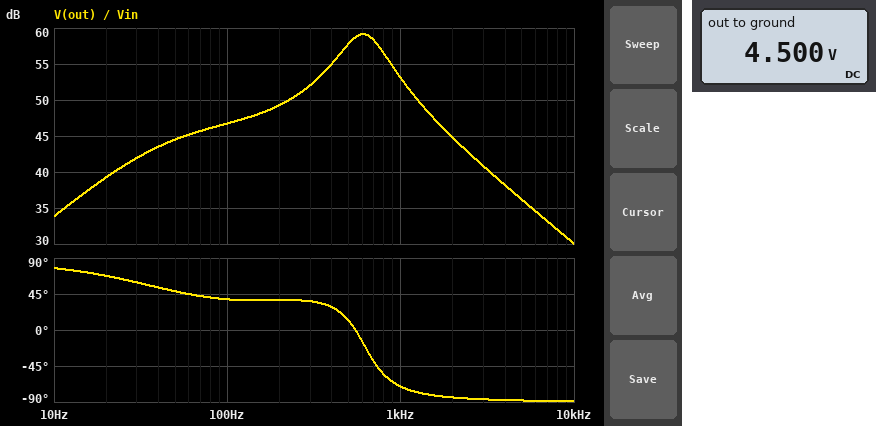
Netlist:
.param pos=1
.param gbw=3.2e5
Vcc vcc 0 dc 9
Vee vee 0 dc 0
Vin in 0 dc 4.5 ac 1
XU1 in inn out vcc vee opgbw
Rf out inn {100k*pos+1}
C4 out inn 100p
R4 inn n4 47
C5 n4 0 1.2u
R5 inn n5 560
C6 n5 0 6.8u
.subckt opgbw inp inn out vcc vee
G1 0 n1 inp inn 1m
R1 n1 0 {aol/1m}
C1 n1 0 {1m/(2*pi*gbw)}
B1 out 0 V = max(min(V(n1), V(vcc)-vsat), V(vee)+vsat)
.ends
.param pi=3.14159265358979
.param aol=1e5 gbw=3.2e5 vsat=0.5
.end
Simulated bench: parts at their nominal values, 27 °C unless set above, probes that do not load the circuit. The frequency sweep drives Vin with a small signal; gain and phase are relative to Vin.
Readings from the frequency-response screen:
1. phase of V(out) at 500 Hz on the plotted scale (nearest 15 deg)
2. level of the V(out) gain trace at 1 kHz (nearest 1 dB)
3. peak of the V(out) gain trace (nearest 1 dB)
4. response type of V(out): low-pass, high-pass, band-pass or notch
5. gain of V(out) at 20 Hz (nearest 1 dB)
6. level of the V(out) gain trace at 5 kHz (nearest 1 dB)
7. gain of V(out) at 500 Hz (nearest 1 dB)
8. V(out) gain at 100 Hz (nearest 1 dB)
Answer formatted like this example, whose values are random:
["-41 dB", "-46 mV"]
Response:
["15 deg", "53 dB", "59 dB", "band-pass", "39 dB", "36 dB", "58 dB", "47 dB"]
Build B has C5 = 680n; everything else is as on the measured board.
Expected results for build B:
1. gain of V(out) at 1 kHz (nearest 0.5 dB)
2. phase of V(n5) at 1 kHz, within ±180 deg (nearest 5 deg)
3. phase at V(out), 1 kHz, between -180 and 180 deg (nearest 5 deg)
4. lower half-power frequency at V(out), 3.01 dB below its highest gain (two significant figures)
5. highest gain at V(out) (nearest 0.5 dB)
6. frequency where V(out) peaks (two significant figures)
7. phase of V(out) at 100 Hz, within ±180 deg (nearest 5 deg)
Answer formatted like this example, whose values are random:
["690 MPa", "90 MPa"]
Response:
["54.5 dB", "165 deg", "-50 deg", "540 Hz", "56.0 dB", "800 Hz", "30 deg"]
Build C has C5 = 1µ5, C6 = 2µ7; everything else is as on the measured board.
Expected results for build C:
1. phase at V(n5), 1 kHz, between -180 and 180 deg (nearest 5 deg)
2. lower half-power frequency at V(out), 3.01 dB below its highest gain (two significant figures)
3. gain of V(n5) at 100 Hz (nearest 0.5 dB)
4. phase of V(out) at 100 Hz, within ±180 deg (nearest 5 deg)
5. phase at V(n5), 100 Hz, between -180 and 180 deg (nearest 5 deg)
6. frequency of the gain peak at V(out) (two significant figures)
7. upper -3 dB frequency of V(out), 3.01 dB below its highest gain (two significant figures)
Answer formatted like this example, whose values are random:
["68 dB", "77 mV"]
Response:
["150 deg", "390 Hz", "-2.5 dB", "60 deg", "-45 deg", "530 Hz", "710 Hz"]
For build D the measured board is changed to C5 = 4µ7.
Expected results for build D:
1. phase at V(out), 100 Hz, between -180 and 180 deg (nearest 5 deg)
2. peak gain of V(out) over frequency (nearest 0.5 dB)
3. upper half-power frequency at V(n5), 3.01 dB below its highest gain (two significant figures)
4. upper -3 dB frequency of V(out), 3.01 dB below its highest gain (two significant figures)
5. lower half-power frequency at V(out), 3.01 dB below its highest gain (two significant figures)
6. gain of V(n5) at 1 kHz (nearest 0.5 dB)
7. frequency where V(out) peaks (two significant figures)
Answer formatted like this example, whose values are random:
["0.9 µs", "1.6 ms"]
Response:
["55 deg", "64.5 dB", "44 Hz", "420 Hz", "220 Hz", "-42.5 dB", "310 Hz"]
